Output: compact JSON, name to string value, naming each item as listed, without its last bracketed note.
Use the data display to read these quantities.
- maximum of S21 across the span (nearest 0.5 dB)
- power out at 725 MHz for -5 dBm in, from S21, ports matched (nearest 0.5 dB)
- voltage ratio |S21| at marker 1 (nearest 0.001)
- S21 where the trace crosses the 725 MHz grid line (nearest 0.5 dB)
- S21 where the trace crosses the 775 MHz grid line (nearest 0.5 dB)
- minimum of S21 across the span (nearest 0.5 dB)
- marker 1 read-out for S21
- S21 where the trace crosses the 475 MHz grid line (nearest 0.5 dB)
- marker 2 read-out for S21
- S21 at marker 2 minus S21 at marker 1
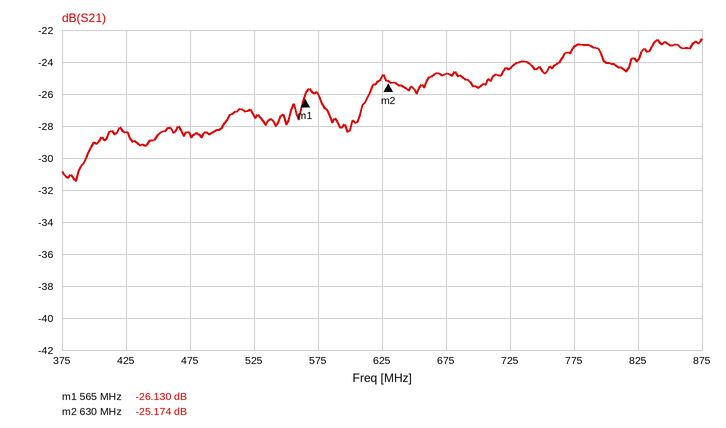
{"maximum of S21 across the span": "-22.5 dB", "power out at 725 MHz for -5 dBm in, from S21, ports matched": "-29.5 dBm", "voltage ratio |S21| at marker 1": "0.049", "S21 where the trace crosses the 725 MHz grid line": "-24.5 dB", "S21 where the trace crosses the 775 MHz grid line": "-23.0 dB", "minimum of S21 across the span": "-31.5 dB", "marker 1 read-out for S21": "-26.130 dB", "S21 where the trace crosses the 475 MHz grid line": "-28.5 dB", "marker 2 read-out for S21": "-25.174 dB", "S21 at marker 2 minus S21 at marker 1": "0.956 dB"}
